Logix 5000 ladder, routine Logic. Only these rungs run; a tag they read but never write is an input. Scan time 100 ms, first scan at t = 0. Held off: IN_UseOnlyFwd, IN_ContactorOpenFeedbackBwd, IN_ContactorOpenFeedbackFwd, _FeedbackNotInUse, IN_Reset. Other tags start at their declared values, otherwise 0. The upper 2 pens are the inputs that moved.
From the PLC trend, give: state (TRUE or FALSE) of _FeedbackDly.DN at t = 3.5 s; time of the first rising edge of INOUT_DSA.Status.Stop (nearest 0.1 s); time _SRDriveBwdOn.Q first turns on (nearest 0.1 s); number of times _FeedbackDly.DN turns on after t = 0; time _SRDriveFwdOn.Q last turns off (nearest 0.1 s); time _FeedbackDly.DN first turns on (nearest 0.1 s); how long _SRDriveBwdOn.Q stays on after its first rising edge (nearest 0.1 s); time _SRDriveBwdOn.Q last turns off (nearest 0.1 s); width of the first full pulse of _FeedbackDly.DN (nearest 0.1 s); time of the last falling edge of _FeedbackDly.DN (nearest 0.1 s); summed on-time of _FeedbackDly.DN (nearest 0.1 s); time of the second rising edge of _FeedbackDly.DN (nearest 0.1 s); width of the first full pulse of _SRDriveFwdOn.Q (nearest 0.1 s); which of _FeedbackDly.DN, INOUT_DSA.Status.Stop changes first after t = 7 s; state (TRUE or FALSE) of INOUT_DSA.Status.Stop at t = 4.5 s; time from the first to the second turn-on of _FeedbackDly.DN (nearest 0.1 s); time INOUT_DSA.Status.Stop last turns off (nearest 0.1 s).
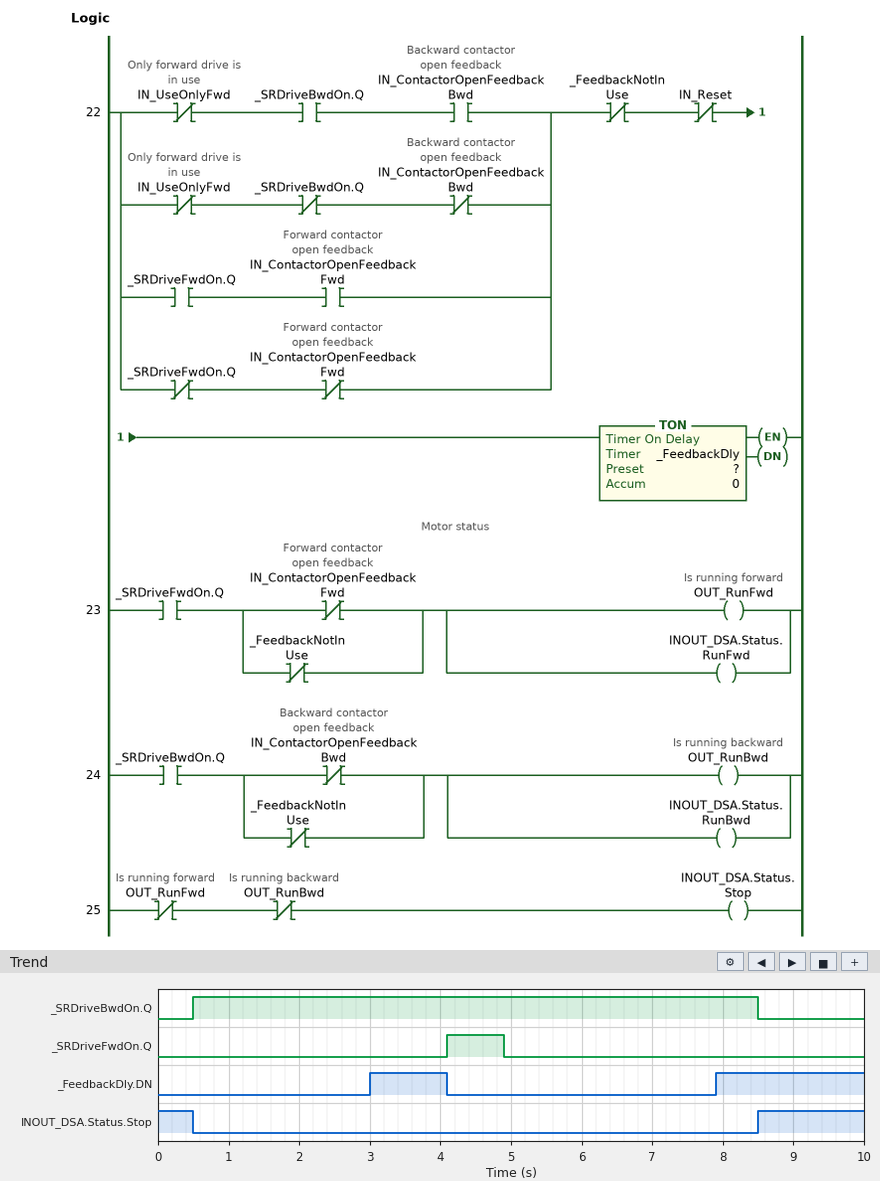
TRUE
8.5 s
0.5 s
2
4.9 s
3.0 s
8.0 s
8.5 s
1.1 s
4.1 s
3.2 s
7.9 s
0.8 s
_FeedbackDly.DN
FALSE
4.9 s
0.5 s
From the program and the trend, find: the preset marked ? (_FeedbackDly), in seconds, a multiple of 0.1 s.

3.0 s
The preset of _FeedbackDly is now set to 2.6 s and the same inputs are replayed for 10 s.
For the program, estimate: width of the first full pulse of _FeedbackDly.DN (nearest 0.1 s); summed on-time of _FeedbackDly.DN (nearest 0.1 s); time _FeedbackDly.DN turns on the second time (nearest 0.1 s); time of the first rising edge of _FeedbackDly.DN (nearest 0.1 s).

1.5 s
4.0 s
7.5 s
2.6 s
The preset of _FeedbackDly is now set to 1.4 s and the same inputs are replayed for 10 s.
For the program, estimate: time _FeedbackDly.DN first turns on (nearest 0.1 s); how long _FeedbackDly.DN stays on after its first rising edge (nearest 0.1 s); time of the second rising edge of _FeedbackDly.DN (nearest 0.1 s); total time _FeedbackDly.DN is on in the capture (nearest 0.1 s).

1.4 s
2.7 s
6.3 s
6.4 s
